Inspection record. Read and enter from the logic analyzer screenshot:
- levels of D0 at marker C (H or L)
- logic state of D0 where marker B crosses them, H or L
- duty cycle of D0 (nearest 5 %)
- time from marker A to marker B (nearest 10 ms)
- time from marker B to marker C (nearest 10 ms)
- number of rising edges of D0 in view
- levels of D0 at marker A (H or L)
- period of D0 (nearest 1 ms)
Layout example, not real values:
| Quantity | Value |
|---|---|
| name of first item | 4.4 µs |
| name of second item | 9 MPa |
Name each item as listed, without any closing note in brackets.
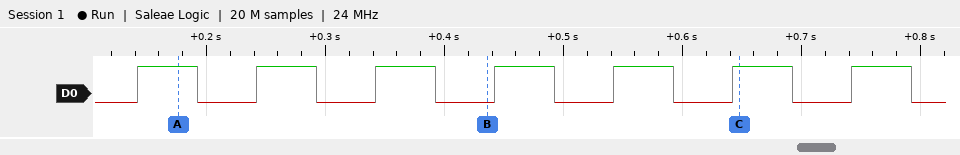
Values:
| Quantity | Value |
|---|---|
| levels of D0 at marker C | D0=H |
| logic state of D0 where marker B crosses them, H or L | D0=L |
| duty cycle of D0 | 50 % |
| time from marker A to marker B | 260 ms |
| time from marker B to marker C | 210 ms |
| number of rising edges of D0 in view | 7 |
| levels of D0 at marker A | D0=H |
| period of D0 | 100 ms |
